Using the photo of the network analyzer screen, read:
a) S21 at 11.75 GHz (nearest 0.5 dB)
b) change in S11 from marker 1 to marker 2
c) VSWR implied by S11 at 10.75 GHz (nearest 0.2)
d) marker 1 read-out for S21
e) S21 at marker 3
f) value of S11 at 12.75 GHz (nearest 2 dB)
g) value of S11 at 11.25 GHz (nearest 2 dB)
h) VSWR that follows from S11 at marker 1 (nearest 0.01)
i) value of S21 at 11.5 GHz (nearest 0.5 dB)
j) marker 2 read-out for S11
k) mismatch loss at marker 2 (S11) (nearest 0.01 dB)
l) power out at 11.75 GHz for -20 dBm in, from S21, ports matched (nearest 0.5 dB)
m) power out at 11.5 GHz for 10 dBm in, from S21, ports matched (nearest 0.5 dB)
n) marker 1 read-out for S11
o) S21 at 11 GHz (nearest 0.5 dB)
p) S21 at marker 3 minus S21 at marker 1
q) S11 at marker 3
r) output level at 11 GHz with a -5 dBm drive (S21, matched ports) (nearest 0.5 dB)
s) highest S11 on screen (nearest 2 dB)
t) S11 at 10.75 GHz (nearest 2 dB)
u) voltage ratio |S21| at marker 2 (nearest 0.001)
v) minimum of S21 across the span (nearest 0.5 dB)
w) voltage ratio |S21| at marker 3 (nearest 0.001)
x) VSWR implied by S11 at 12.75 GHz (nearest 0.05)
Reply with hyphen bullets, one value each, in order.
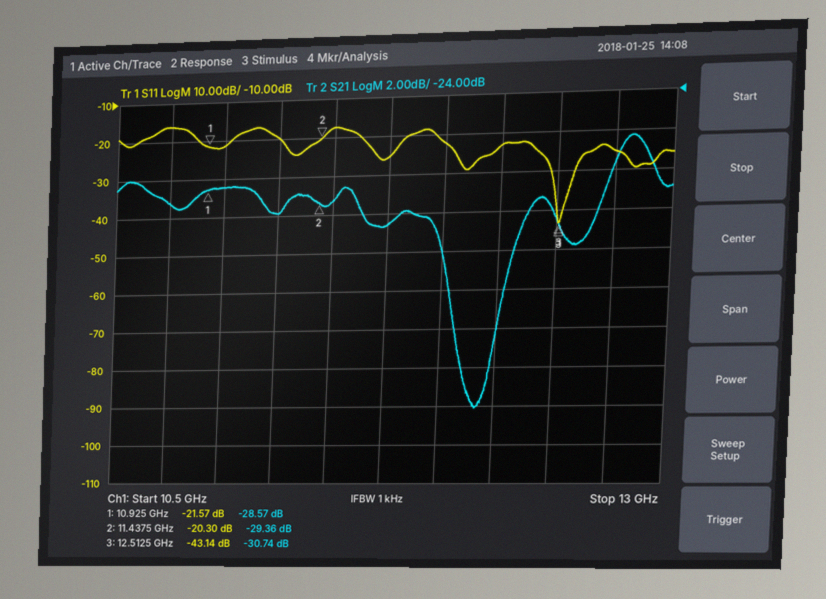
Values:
- -30.5 dB
- 1.27 dB
- 1.4
- -28.57 dB
- -30.74 dB
- -26 dB
- -20 dB
- 1.18
- -29.5 dB
- -20.30 dB
- 0.04 dB
- -50.5 dBm
- -19.5 dBm
- -21.57 dB
- -28.5 dB
- -2.17 dB
- -43.14 dB
- -33.5 dBm
- -16 dB
- -16 dB
- 0.034
- -40.0 dB
- 0.029
- 1.10
